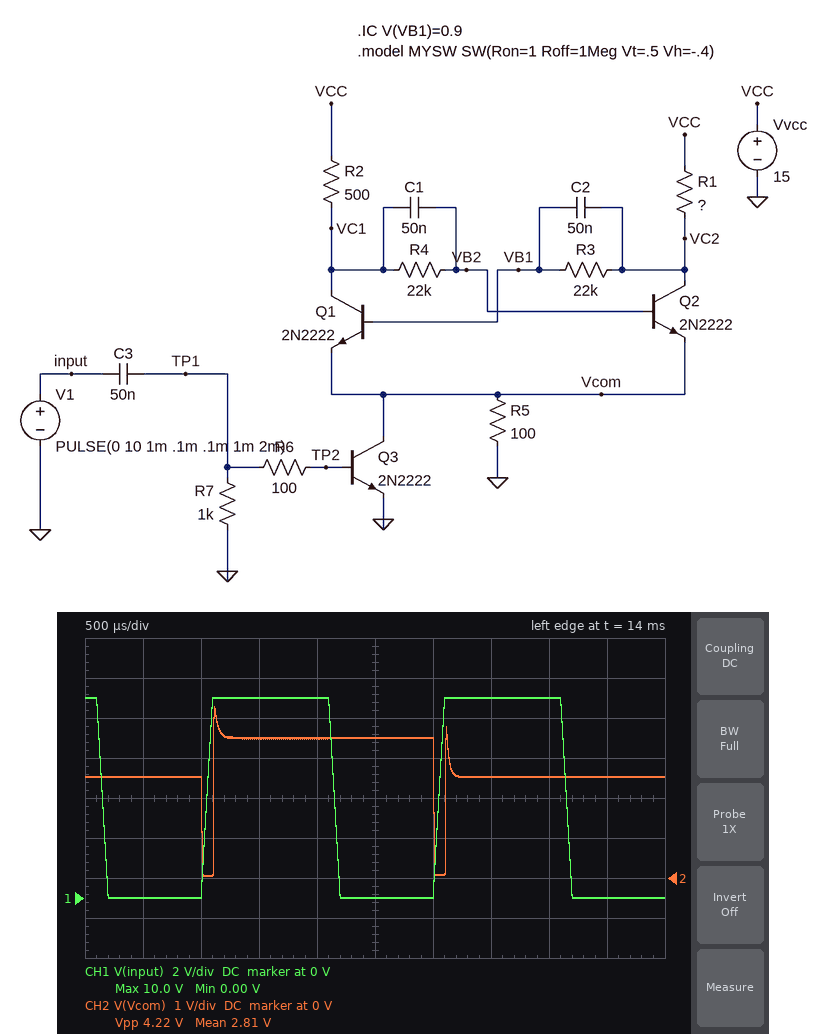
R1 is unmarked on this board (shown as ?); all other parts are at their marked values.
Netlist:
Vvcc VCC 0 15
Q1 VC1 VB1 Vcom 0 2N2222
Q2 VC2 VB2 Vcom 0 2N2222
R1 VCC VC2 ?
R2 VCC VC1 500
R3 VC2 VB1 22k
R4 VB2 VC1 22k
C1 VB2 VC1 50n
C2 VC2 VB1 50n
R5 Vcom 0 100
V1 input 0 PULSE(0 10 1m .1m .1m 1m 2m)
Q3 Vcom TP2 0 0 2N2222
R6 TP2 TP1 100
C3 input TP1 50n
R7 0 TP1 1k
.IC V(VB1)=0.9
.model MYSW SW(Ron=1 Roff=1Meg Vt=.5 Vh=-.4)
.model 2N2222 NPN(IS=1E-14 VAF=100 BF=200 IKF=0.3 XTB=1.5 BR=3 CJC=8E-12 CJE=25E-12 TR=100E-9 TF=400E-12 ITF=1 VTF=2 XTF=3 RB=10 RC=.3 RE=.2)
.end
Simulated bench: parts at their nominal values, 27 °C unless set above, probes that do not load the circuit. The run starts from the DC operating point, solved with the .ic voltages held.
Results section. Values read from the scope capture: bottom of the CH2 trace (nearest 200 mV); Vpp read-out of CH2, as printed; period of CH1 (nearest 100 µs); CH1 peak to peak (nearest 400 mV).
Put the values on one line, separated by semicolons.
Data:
0 V; 4.22 V; 2.0 ms; 10.0 V
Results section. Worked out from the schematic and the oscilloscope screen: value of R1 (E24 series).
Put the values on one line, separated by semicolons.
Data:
330 Ω
